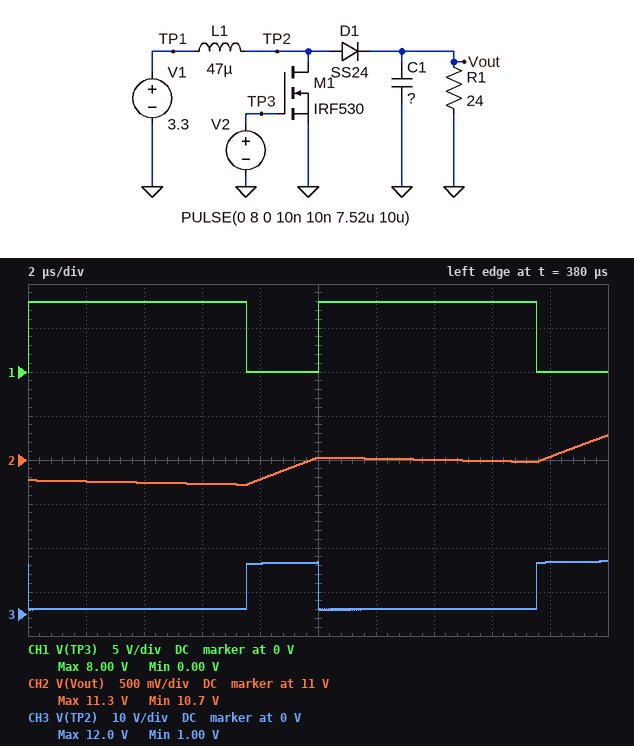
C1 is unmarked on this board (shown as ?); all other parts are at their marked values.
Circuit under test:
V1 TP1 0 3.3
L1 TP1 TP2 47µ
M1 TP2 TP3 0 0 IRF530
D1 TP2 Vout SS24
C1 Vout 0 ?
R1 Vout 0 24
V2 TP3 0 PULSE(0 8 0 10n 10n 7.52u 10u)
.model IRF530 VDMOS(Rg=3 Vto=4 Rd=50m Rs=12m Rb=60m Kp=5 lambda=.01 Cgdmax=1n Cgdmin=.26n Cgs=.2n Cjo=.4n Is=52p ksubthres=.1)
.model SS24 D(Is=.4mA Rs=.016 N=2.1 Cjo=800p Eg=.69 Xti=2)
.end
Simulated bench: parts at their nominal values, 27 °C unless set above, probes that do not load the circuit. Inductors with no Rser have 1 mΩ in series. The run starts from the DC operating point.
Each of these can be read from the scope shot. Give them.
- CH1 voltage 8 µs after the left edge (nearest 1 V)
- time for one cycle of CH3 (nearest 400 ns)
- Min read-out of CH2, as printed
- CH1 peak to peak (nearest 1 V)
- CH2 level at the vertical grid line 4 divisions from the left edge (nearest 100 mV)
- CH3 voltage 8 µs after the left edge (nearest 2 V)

0 V
10.0 µs
10.7 V
8 V
10.8 V
12 V
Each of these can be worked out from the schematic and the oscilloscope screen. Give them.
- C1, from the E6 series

68 µF
